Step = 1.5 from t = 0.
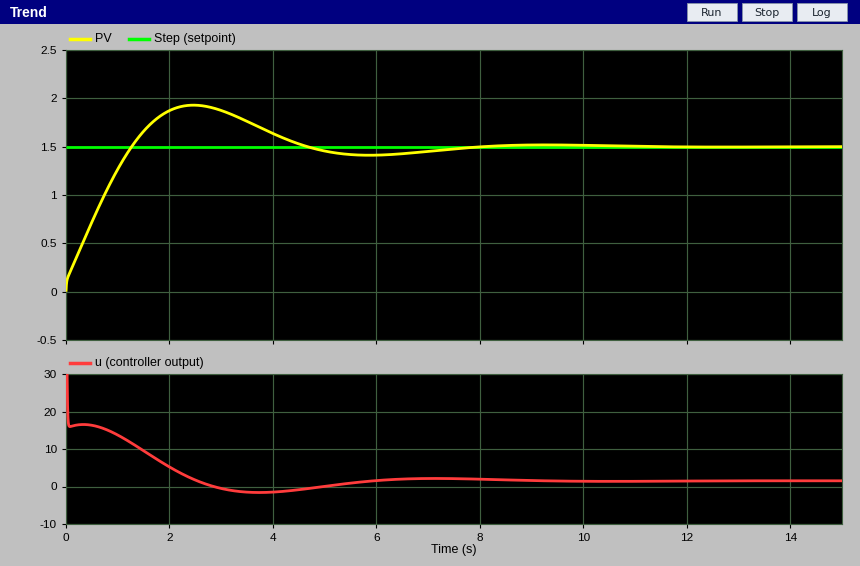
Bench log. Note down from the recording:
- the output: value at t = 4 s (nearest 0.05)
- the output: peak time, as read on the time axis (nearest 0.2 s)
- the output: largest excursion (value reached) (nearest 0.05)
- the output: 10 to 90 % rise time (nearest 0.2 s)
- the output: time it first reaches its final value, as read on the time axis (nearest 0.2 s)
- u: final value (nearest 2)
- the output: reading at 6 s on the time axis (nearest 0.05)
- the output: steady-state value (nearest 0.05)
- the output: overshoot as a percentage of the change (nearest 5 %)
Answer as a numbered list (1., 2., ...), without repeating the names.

1. 1.65
2. 2.4 s
3. 1.95
4. 1.0 s
5. 1.2 s
6. 2
7. 1.40
8. 1.50
9. 30 %
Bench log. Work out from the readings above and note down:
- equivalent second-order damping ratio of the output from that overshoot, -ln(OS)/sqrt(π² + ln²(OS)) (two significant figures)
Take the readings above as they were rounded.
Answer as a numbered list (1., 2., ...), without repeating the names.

1. 0.36
